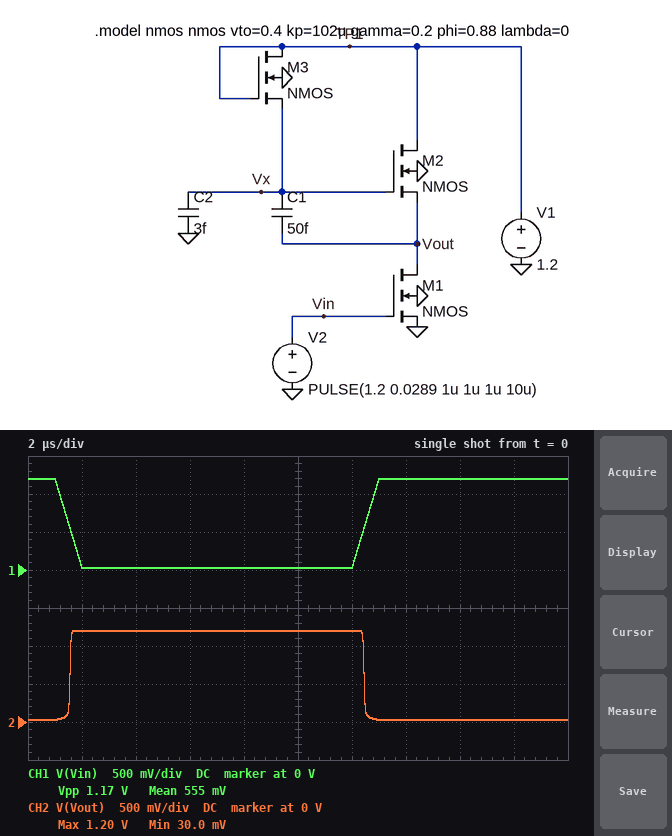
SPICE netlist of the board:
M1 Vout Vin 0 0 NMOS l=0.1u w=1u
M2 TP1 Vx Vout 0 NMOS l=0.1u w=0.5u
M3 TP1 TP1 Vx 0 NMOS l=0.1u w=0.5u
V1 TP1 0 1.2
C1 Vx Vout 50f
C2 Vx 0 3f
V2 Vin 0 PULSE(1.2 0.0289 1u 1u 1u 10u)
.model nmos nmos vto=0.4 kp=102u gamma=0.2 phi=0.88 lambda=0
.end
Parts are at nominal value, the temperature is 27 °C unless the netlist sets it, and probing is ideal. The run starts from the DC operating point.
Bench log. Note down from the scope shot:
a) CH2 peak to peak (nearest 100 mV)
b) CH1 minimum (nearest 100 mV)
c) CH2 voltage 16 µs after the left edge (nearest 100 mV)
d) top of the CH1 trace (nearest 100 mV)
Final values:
1.2 V
0 V
0 V
1.2 V
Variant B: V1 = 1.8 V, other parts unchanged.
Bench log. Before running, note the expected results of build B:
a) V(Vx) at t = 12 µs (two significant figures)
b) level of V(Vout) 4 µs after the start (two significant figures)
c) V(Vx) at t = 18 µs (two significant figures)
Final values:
2.8 V
1.8 V
1.3 V
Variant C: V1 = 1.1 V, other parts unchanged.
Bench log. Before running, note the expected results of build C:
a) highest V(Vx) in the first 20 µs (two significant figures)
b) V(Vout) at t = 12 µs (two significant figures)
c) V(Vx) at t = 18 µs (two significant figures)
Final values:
1.7 V
1.1 V
640 mV
